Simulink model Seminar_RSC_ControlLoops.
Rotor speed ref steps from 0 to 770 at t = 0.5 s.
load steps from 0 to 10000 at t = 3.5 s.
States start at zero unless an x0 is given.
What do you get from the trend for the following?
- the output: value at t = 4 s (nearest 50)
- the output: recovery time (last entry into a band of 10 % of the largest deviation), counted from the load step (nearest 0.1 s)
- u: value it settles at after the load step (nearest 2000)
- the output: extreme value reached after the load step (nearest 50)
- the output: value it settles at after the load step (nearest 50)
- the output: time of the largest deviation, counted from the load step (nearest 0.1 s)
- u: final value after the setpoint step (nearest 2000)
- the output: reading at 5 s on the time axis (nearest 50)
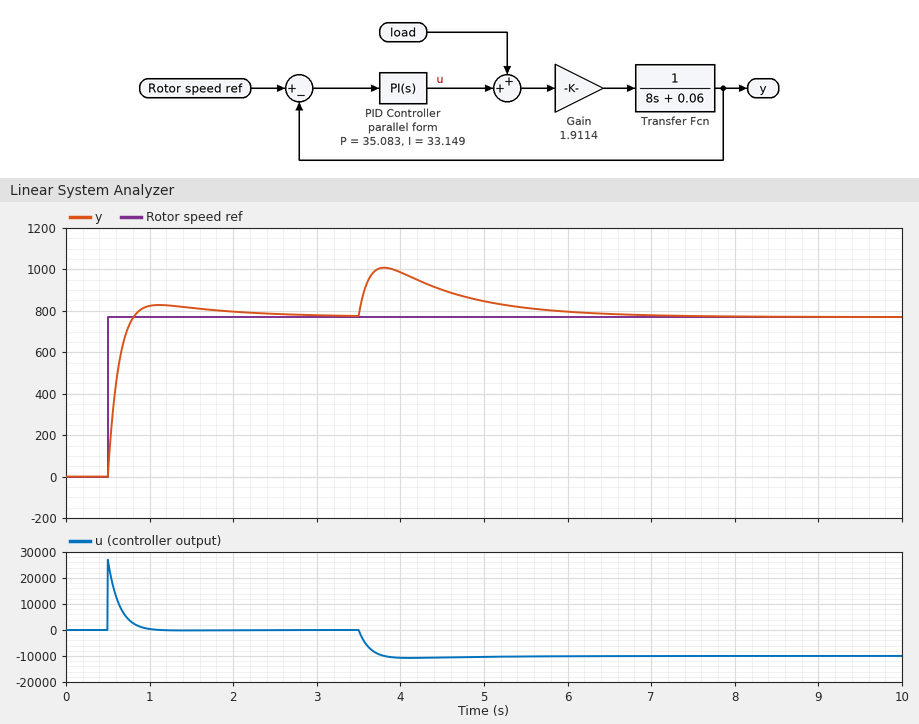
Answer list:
1000
2.6 s
-10000
1000
750
0.3 s
0
850
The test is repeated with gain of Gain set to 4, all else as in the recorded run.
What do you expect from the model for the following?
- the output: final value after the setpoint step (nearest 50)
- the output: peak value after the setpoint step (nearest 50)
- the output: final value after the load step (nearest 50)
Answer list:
750
800
750
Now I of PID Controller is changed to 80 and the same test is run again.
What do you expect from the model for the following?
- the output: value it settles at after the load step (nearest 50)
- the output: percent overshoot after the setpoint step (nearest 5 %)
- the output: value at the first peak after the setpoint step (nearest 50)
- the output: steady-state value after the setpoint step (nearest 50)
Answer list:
750
15 %
900
750
